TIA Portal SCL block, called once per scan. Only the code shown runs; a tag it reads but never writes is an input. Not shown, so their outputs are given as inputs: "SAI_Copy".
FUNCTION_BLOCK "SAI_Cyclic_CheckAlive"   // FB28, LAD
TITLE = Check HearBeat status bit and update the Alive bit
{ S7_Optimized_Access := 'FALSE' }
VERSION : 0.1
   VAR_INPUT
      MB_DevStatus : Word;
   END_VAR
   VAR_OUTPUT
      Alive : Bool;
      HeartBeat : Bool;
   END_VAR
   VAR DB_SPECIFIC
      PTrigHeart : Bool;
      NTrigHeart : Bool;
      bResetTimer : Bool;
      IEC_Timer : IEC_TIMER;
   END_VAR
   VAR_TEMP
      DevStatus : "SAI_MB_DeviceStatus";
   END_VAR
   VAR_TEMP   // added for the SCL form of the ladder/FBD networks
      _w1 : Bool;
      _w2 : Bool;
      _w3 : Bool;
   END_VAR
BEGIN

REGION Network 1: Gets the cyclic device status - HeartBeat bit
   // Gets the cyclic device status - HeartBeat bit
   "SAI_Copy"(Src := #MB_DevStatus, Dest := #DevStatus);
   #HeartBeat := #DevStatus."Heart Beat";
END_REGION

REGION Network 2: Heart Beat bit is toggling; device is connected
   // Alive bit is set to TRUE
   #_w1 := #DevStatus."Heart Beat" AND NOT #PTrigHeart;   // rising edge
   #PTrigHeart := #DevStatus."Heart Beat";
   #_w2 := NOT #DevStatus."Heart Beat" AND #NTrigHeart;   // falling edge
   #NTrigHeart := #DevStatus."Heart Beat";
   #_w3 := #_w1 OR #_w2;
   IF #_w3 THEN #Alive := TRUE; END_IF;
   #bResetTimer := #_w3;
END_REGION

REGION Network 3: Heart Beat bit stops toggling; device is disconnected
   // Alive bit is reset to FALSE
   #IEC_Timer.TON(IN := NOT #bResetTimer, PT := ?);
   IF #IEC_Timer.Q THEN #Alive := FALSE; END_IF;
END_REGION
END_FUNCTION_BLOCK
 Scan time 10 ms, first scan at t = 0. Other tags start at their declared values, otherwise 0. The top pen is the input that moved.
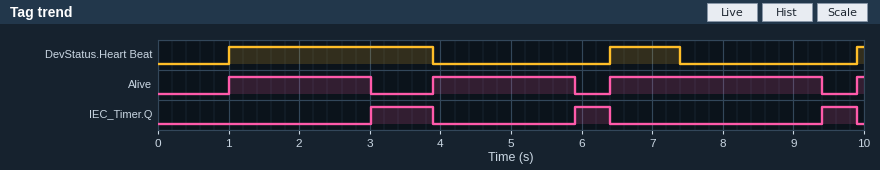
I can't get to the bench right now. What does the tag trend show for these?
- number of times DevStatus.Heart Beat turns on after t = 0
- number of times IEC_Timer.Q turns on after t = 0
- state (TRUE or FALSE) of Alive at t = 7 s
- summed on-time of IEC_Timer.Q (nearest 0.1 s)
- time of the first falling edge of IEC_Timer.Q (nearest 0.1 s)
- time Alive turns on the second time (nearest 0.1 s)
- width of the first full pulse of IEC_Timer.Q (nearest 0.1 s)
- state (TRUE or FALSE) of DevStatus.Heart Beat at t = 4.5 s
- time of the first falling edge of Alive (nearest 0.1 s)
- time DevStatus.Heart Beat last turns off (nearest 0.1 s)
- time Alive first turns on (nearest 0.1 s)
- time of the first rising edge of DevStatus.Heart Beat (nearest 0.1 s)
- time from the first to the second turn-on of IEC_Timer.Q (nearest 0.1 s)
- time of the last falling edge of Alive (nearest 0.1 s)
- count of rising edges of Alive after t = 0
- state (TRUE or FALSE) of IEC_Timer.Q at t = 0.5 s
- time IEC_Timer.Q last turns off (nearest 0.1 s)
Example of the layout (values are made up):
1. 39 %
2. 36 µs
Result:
1. 3
2. 3
3. TRUE
4. 1.9 s
5. 3.9 s
6. 3.9 s
7. 0.9 s
8. FALSE
9. 3.0 s
10. 7.4 s
11. 1.0 s
12. 1.0 s
13. 2.9 s
14. 9.4 s
15. 4
16. FALSE
17. 9.9 s
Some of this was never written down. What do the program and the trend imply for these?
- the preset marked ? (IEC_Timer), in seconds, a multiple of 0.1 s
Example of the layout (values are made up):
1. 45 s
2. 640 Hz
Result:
1. 2.0 s
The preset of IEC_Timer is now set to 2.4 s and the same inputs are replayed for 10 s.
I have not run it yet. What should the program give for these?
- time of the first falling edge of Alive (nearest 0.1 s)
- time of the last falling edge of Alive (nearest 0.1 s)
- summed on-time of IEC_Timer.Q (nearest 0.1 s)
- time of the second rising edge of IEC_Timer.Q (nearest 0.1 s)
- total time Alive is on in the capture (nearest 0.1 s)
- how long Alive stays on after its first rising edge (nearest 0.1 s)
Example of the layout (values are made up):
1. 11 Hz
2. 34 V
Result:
1. 3.4 s
2. 9.8 s
3. 0.7 s
4. 6.3 s
5. 8.3 s
6. 2.4 s
